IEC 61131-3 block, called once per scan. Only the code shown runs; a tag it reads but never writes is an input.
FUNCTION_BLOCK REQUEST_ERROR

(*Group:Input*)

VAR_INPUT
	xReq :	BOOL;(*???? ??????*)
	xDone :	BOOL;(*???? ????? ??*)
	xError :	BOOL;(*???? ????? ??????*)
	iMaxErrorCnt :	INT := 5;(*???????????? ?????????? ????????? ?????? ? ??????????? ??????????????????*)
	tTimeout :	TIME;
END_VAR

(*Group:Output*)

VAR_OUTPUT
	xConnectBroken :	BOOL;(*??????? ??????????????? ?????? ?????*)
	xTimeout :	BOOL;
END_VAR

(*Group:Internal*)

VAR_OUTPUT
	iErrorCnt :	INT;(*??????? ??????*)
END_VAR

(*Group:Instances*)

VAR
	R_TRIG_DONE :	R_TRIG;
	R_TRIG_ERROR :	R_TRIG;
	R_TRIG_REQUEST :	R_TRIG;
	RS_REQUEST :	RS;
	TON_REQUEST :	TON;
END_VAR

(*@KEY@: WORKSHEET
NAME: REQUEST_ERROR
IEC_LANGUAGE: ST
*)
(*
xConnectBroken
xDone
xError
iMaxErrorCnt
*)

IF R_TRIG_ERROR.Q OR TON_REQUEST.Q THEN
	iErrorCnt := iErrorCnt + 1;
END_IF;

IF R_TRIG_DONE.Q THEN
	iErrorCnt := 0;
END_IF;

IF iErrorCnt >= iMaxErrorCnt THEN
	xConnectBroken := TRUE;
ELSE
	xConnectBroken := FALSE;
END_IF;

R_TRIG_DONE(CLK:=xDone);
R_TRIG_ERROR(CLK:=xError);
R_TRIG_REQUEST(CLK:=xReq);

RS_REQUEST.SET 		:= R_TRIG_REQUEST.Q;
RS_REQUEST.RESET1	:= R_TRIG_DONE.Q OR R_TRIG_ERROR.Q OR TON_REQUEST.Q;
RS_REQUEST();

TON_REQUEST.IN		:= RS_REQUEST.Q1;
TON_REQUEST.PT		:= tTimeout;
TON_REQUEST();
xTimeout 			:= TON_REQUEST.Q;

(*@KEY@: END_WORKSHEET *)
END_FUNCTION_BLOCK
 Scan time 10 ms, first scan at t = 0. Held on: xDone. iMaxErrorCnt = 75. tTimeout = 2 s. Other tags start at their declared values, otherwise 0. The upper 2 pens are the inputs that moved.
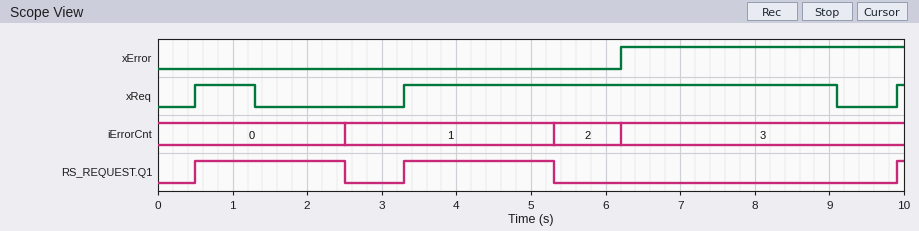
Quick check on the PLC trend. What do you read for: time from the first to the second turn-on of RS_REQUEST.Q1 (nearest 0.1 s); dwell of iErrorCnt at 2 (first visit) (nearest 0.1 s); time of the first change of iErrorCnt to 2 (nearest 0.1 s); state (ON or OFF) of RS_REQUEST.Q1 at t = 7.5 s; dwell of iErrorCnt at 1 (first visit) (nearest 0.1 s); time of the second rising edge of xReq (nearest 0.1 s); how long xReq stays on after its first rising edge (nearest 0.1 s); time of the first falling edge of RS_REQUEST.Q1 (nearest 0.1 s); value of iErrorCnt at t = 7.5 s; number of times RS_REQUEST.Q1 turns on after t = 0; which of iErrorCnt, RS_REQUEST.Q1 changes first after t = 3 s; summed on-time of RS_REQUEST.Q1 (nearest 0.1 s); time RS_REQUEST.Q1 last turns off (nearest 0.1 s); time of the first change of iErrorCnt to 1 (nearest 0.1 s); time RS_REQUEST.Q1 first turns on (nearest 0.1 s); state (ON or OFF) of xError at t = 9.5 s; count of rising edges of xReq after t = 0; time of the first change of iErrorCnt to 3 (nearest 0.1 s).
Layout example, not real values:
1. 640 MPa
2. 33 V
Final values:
1. 2.8 s
2. 0.9 s
3. 5.3 s
4. OFF
5. 2.8 s
6. 3.3 s
7. 0.8 s
8. 2.5 s
9. 3
10. 3
11. RS_REQUEST.Q1
12. 4.1 s
13. 5.3 s
14. 2.5 s
15. 0.5 s
16. ON
17. 3
18. 6.2 s
